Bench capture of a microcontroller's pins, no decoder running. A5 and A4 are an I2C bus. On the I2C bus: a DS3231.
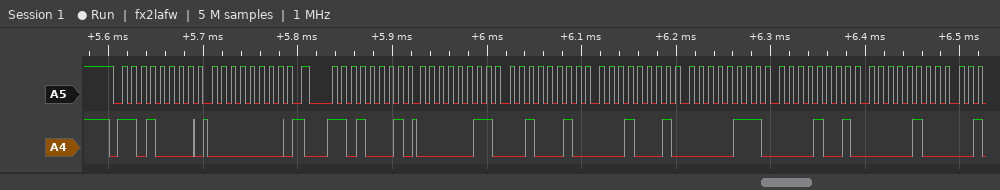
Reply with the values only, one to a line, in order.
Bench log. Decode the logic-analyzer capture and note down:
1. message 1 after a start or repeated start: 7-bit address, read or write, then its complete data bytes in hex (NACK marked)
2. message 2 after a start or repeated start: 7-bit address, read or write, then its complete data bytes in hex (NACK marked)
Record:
0x68 write: 00
0x68 read: 03 22 11 07 09 04
